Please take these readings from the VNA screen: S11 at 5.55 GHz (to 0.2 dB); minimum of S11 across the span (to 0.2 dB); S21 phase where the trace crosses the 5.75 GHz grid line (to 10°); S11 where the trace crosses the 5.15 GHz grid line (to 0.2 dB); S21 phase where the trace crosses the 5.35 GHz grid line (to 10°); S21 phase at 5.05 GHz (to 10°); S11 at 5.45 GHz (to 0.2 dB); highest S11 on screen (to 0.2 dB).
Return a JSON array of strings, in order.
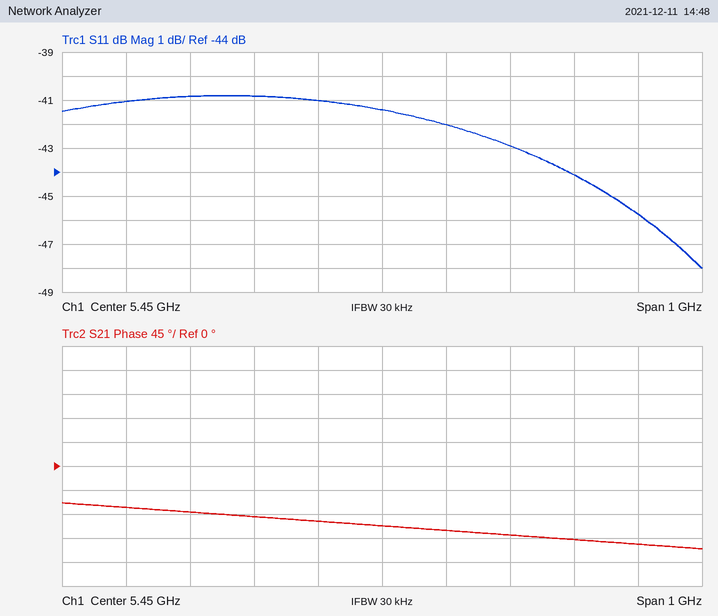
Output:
["-42.0 dB", "-48.0 dB", "-140°", "-40.8 dB", "-100°", "-80°", "-41.4 dB", "-40.8 dB"]
